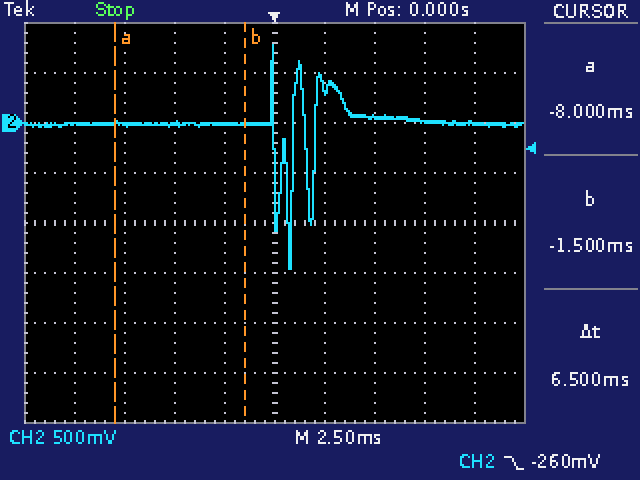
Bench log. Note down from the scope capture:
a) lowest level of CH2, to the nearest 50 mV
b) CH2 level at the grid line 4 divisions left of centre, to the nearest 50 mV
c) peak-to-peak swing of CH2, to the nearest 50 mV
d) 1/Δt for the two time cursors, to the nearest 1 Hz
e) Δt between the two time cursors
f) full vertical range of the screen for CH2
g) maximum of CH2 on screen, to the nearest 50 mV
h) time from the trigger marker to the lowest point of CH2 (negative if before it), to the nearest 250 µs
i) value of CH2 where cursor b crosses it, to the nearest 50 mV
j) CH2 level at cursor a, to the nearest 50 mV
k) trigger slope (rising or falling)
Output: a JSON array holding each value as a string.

["-1.45 V", "0 mV", "2.25 V", "154 Hz", "6.5 ms", "4 V", "800 mV", "+750 µs", "0 mV", "0 mV", "falling"]
